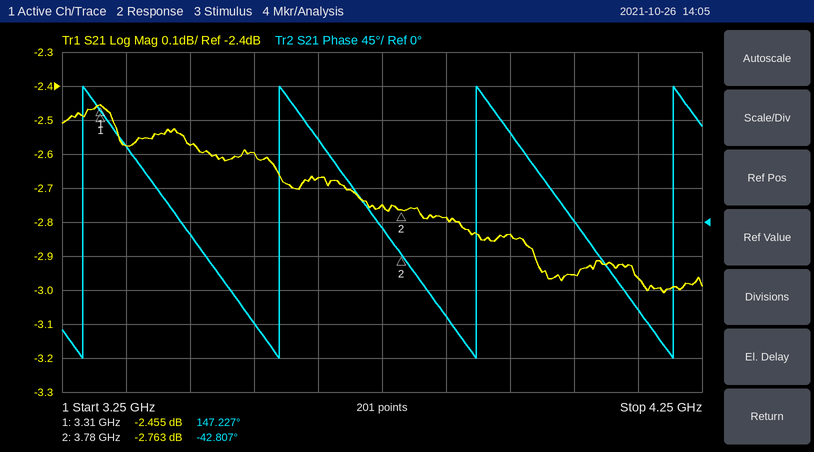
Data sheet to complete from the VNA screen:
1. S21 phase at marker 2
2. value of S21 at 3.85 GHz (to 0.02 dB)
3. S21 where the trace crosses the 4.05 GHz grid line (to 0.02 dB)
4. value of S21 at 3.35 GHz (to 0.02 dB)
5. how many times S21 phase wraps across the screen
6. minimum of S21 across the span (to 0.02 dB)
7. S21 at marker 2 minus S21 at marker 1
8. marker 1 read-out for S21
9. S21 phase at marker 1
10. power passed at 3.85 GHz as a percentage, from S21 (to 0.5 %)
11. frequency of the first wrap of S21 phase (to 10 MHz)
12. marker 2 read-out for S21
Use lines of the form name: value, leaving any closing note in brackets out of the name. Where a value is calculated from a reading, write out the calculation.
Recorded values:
S21 phase at marker 2: -42.807°
value of S21 at 3.85 GHz: -2.78 dB
S21 where the trace crosses the 4.05 GHz grid line: -2.96 dB
value of S21 at 3.35 GHz: -2.58 dB
how many times S21 phase wraps across the screen: 4
minimum of S21 across the span: -3.00 dB
S21 at marker 2 minus S21 at marker 1: -2.763 − (-2.455) = -0.308 dB
marker 1 read-out for S21: -2.455 dB
S21 phase at marker 1: 147.227°
power passed at 3.85 GHz as a percentage, from S21: 10^(-2.78/10) ≈ 52.7 %, so 52.5 % to the nearest 0.5 %
frequency of the first wrap of S21 phase: 3.28 GHz
marker 2 read-out for S21: -2.763 dB
